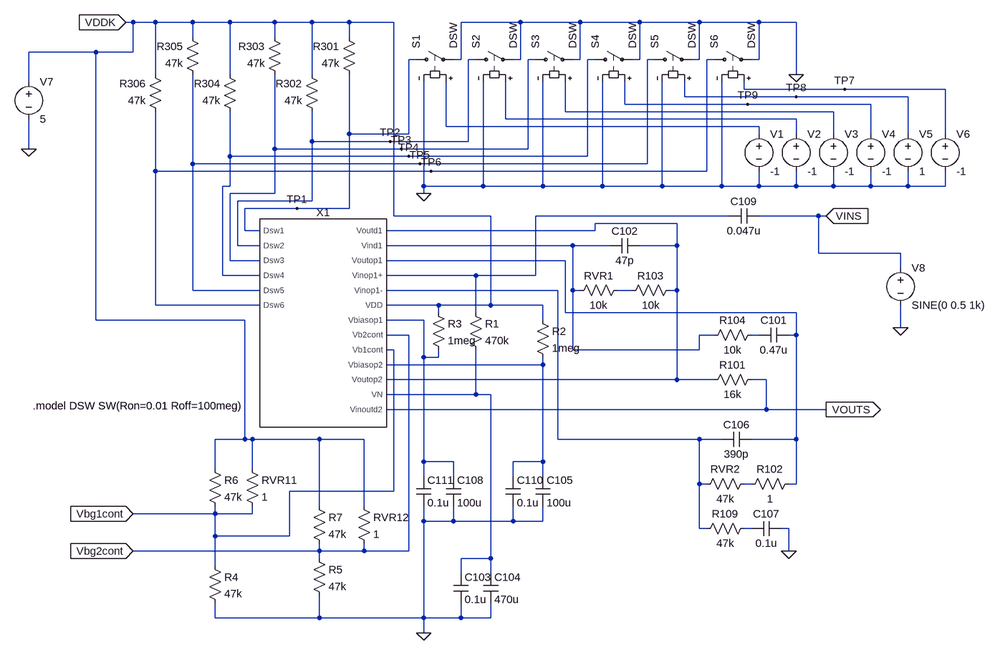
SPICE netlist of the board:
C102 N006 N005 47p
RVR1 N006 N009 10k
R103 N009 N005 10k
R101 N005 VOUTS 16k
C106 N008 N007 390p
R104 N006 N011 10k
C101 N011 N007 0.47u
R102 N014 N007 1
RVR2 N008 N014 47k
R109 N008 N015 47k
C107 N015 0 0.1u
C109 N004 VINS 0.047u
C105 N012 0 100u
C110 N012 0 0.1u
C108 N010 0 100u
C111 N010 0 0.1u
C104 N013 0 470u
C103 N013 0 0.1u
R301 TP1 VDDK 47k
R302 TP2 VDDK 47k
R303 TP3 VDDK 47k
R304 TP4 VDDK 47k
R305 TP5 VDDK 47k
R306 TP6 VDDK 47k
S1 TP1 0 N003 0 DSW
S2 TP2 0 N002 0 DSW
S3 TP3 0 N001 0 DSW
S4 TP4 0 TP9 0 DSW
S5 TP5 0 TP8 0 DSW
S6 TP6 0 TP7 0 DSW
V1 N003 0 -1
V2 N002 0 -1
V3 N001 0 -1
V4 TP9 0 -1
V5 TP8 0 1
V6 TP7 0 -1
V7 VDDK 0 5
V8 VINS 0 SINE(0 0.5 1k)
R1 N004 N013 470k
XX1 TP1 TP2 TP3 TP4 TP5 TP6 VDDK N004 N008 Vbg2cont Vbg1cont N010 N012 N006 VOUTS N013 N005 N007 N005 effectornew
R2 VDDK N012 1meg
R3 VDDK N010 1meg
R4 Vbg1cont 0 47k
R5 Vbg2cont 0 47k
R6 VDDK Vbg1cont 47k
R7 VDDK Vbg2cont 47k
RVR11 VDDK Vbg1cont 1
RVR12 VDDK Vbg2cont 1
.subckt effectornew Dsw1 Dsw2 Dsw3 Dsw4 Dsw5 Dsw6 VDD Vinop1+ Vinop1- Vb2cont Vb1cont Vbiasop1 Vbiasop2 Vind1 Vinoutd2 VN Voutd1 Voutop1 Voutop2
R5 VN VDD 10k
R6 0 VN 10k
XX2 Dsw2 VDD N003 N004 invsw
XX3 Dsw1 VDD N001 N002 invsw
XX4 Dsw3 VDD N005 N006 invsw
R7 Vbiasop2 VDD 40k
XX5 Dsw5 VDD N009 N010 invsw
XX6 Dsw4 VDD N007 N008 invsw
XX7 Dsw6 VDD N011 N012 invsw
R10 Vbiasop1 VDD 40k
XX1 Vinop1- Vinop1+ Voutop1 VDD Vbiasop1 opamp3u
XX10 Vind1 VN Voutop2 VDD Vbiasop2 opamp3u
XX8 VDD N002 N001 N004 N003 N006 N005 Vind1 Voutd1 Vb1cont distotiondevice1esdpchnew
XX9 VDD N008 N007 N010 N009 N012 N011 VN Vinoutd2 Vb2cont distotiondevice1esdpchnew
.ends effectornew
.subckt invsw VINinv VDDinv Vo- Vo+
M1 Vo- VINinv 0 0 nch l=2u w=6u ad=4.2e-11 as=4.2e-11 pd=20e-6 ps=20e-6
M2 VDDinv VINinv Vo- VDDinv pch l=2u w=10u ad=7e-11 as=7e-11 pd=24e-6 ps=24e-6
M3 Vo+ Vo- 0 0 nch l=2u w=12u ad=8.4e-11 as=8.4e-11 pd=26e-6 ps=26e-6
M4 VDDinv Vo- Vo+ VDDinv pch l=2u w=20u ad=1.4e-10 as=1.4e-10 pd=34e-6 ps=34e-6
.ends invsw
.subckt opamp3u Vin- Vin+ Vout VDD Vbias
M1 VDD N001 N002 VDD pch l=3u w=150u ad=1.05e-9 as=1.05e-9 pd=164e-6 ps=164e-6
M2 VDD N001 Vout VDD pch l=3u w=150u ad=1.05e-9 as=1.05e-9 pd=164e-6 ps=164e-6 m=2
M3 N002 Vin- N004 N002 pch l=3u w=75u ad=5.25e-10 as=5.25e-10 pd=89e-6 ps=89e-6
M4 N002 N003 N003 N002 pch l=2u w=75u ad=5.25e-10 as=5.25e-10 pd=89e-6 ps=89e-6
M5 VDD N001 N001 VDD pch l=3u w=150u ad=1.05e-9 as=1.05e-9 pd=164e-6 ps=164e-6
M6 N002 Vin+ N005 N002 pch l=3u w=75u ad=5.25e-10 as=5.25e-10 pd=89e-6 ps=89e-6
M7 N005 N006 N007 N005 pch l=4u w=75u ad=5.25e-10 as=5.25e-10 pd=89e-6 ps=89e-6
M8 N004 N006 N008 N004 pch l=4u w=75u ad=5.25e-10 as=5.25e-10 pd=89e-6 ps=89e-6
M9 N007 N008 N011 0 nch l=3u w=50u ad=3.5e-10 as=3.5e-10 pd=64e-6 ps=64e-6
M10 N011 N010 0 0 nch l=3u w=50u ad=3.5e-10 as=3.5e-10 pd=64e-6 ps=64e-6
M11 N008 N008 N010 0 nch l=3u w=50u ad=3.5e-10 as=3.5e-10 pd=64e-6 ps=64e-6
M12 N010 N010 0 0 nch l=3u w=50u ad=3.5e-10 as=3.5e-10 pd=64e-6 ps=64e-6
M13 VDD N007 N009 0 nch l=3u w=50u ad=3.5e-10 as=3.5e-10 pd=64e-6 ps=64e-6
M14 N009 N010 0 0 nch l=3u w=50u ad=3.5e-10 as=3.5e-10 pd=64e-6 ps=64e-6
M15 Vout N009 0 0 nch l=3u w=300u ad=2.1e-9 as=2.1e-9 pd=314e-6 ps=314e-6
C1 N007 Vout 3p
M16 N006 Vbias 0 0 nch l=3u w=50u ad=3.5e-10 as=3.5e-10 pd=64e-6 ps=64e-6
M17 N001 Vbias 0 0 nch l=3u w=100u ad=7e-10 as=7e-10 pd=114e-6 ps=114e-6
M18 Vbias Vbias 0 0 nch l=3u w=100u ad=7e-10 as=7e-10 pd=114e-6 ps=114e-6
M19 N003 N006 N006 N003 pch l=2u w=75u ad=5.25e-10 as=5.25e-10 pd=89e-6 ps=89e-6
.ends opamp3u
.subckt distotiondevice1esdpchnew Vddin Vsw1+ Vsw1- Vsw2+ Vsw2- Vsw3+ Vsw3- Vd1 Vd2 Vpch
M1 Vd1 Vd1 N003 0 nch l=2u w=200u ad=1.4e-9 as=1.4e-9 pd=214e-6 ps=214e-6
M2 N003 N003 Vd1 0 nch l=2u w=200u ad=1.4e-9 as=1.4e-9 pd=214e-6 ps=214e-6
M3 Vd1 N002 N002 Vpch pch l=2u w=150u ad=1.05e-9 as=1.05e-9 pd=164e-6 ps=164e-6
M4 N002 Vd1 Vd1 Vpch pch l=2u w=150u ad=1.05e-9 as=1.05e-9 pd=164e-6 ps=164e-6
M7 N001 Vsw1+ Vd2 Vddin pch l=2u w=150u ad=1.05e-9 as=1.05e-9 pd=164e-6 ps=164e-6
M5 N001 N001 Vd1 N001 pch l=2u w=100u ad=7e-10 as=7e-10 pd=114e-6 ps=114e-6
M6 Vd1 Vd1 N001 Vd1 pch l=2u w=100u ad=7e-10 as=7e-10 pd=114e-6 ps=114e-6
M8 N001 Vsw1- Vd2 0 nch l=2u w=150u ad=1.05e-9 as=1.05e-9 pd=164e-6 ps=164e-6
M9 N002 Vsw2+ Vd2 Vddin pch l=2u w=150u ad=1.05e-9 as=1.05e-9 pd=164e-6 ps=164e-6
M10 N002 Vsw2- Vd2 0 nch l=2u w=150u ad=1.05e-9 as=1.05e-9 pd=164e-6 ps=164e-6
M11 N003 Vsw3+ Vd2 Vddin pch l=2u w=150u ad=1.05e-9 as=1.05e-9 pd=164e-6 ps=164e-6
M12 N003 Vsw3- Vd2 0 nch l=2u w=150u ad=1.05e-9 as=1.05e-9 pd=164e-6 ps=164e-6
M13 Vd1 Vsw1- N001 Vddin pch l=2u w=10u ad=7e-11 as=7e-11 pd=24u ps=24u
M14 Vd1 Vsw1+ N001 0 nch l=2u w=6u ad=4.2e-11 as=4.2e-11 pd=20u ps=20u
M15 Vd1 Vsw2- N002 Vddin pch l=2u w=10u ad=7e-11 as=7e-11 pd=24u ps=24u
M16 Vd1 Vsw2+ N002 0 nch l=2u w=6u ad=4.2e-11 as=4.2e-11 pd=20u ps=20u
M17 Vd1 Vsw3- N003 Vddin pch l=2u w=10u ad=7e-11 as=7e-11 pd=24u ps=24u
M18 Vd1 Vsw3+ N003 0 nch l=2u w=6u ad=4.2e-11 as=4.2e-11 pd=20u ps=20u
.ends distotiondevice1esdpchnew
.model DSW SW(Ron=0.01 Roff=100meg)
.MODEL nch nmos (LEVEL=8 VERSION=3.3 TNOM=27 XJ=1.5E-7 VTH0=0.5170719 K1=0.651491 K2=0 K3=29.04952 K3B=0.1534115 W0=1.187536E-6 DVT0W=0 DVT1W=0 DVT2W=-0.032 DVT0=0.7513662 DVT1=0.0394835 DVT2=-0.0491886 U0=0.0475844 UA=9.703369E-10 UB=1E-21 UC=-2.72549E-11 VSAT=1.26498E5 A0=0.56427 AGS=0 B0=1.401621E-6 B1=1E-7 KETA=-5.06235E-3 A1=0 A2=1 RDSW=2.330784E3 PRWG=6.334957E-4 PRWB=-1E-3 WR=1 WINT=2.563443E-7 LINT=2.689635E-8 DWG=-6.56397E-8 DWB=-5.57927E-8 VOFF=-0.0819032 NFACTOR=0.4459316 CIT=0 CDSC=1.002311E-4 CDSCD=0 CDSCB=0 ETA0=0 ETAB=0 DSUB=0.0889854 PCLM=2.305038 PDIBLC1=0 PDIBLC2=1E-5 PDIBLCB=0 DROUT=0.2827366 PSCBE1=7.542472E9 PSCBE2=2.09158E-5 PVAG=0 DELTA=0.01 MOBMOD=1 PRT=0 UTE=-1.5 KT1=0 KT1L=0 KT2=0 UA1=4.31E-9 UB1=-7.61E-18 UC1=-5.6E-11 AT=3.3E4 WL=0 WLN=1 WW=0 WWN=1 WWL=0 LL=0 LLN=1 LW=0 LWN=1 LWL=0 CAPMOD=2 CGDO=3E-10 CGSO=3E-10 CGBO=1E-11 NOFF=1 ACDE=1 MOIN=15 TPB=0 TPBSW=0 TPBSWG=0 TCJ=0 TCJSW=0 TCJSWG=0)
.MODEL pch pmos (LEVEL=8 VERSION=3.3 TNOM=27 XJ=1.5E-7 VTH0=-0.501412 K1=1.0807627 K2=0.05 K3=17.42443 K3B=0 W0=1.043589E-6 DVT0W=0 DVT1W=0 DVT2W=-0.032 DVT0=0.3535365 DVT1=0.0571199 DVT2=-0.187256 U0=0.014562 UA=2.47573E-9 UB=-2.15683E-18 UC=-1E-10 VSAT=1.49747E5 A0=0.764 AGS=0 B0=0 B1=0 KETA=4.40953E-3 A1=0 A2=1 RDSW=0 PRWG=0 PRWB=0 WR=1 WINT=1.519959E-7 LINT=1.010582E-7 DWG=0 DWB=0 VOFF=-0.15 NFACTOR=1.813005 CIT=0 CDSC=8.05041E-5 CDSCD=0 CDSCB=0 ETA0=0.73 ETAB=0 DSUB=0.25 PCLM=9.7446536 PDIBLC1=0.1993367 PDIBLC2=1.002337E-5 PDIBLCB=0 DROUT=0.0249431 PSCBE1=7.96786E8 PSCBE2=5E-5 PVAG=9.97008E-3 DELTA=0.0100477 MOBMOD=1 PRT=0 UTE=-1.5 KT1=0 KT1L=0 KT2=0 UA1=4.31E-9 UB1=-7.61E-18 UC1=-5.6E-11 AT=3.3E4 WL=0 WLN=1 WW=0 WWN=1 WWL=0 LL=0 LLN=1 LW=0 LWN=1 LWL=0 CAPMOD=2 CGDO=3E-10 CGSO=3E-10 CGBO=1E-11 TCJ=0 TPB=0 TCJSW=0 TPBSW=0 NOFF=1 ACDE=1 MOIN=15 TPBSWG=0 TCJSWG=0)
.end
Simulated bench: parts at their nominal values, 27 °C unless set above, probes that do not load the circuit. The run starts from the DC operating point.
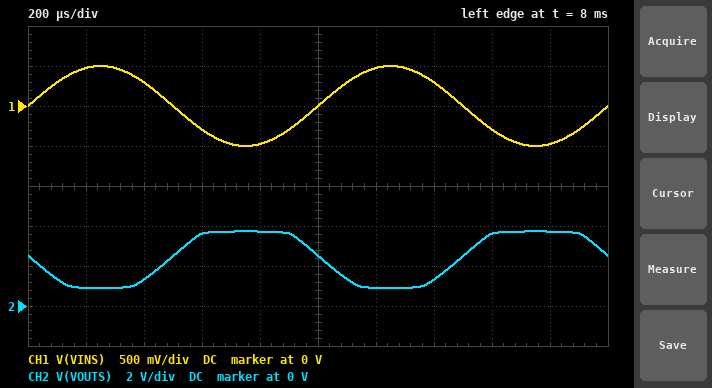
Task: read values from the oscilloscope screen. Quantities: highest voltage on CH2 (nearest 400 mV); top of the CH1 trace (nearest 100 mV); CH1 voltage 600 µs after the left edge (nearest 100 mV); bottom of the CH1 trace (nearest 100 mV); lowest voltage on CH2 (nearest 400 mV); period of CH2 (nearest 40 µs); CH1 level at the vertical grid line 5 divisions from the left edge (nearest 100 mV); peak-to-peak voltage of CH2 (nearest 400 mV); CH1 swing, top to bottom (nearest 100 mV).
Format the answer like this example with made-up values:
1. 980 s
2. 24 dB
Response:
1. 3.6 V
2. 500 mV
3. -300 mV
4. -500 mV
5. 800 mV
6. 1.00 ms
7. 0 V
8. 2.8 V
9. 1.0 V
